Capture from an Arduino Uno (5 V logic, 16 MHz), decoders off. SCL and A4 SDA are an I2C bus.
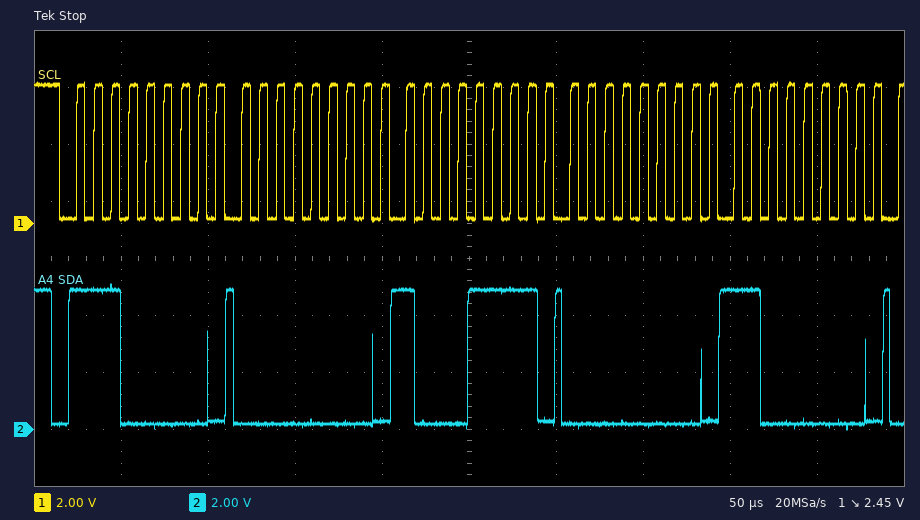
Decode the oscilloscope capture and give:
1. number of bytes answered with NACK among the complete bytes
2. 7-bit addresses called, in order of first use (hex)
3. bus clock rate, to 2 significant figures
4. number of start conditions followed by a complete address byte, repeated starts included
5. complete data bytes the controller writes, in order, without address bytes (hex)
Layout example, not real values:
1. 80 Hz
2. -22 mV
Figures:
1. 0
2. 0x70
3. 100 kHz
4. 1
5. 00 8F 00 C0
